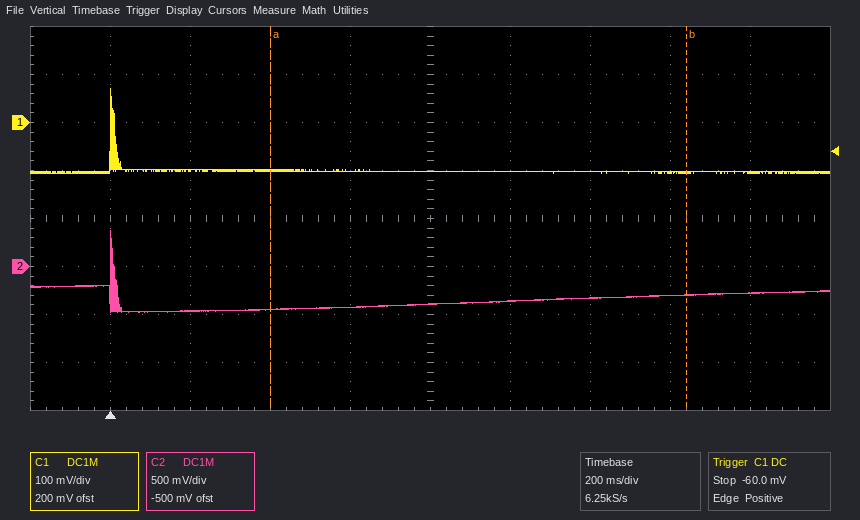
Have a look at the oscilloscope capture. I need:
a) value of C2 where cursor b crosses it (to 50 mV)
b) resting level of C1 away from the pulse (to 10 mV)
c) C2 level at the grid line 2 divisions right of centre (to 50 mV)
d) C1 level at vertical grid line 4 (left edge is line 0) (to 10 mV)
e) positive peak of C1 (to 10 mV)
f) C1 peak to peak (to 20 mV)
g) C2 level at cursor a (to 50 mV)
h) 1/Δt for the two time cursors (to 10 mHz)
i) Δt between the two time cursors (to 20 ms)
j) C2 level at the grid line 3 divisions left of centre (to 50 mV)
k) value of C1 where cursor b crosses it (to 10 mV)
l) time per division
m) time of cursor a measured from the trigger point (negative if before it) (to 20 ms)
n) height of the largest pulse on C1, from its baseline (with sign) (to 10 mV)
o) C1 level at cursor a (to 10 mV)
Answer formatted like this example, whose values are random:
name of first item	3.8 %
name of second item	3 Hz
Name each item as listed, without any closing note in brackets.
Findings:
value of C2 where cursor b crosses it	-300 mV
resting level of C1 away from the pulse	-100 mV
C2 level at the grid line 2 divisions right of centre	-350 mV
C1 level at vertical grid line 4 (left edge is line 0)	-100 mV
positive peak of C1	70 mV
C1 peak to peak	180 mV
C2 level at cursor a	-450 mV
1/Δt for the two time cursors	960 mHz
Δt between the two time cursors	1.04 s
C2 level at the grid line 3 divisions left of centre	-450 mV
value of C1 where cursor b crosses it	-100 mV
time per division	200 ms
time of cursor a measured from the trigger point (negative if before it)	+400 ms
height of the largest pulse on C1, from its baseline (with sign)	+170 mV
C1 level at cursor a	-100 mV
